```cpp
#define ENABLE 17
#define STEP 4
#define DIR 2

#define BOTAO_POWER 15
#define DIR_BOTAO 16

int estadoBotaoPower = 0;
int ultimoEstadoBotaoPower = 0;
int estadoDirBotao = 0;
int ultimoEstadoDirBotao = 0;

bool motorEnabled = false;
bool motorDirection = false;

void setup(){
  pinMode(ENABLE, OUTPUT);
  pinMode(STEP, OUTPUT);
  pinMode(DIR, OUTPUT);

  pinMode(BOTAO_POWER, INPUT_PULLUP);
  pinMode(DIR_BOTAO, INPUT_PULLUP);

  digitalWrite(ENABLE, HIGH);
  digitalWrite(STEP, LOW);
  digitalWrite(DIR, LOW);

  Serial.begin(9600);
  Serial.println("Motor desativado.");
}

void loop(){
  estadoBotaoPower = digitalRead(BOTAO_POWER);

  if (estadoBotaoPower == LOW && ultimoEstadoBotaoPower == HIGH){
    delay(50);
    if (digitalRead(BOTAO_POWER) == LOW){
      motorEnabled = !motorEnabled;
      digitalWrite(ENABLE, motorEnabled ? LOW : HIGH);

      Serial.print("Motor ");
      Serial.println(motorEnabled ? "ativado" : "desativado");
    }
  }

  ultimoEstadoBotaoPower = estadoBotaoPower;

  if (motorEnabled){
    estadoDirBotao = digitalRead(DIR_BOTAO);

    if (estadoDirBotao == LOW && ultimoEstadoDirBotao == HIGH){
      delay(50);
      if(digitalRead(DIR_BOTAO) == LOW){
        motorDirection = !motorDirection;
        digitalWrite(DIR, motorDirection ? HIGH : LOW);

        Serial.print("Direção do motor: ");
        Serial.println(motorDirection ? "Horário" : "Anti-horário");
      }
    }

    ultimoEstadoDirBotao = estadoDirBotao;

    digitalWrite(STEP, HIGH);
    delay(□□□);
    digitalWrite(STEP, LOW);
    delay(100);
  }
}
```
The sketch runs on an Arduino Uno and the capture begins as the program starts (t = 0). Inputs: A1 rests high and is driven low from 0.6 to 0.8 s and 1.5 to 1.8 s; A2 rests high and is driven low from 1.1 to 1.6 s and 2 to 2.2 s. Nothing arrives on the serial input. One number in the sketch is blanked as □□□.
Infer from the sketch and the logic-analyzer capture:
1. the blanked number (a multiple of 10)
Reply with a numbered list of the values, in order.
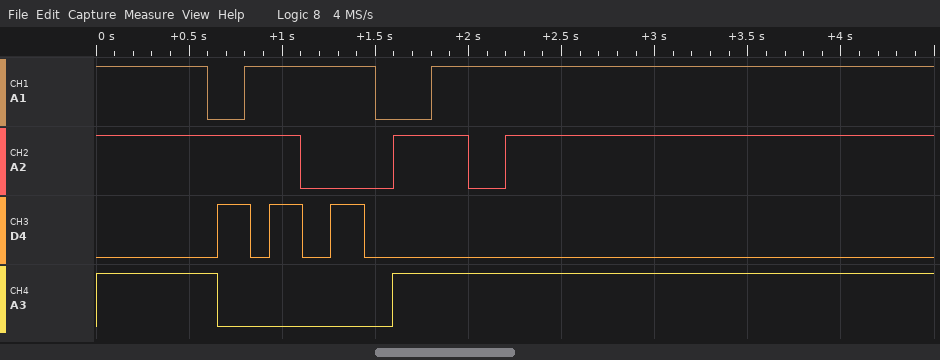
1. 180
